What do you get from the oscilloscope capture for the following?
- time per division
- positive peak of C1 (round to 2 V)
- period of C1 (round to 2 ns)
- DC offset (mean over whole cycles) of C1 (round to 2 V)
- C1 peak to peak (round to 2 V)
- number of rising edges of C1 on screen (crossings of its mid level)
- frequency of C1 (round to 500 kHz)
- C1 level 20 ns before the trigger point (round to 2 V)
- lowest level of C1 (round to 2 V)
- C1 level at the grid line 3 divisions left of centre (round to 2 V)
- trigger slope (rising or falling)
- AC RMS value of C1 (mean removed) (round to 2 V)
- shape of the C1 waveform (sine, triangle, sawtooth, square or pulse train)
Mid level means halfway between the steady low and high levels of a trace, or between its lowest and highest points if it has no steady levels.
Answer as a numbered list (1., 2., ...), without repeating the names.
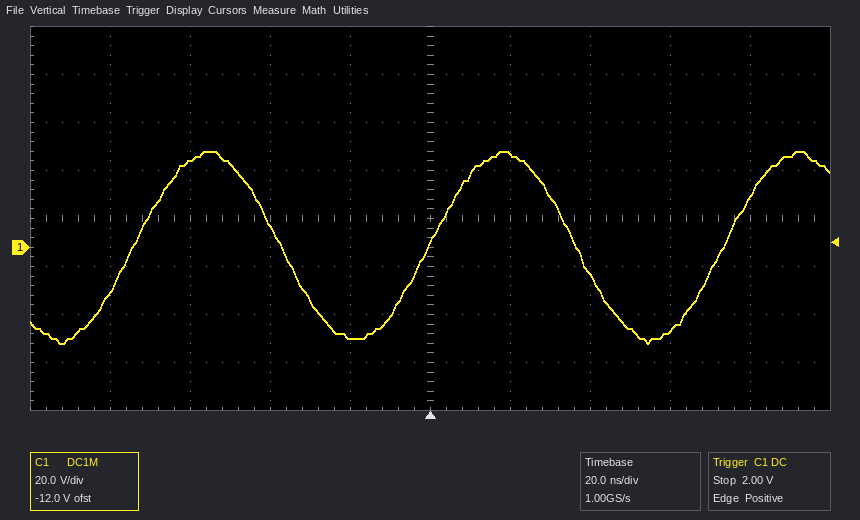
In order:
1. 20 ns
2. 40 V
3. 74 ns
4. 0 V
5. 80 V
6. 3
7. 13.5 MHz
8. -38 V
9. -40 V
10. 36 V
11. rising
12. 28 V
13. sine
